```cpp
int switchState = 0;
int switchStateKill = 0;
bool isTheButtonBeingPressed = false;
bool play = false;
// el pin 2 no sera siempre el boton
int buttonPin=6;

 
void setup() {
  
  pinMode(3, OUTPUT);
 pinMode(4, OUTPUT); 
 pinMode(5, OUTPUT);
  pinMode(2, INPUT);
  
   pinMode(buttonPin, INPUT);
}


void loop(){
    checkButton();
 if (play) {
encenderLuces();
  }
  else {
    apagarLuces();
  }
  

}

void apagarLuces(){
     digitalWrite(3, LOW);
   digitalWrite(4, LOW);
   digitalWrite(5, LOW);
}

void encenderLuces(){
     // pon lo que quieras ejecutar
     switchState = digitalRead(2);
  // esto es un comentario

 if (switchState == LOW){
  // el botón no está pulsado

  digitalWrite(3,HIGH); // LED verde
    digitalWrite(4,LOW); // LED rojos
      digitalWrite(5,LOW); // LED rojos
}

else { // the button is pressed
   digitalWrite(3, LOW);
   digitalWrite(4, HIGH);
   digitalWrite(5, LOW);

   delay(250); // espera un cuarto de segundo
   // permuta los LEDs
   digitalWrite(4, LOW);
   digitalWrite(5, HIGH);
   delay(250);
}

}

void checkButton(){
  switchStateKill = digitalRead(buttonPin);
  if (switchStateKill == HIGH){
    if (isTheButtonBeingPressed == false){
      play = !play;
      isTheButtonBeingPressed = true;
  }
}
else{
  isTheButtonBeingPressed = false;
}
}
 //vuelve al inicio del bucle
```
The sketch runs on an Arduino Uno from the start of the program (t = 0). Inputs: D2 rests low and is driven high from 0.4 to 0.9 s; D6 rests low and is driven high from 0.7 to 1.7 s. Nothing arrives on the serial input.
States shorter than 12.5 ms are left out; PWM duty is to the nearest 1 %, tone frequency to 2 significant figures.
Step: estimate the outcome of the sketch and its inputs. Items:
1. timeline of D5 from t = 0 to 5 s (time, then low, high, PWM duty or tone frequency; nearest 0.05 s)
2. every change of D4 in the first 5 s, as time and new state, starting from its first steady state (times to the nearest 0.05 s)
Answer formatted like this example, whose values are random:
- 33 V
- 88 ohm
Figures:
- 0 s low; 0.95 s high; 1.2 s low
- 0 s low; 0.7 s high; 0.95 s low
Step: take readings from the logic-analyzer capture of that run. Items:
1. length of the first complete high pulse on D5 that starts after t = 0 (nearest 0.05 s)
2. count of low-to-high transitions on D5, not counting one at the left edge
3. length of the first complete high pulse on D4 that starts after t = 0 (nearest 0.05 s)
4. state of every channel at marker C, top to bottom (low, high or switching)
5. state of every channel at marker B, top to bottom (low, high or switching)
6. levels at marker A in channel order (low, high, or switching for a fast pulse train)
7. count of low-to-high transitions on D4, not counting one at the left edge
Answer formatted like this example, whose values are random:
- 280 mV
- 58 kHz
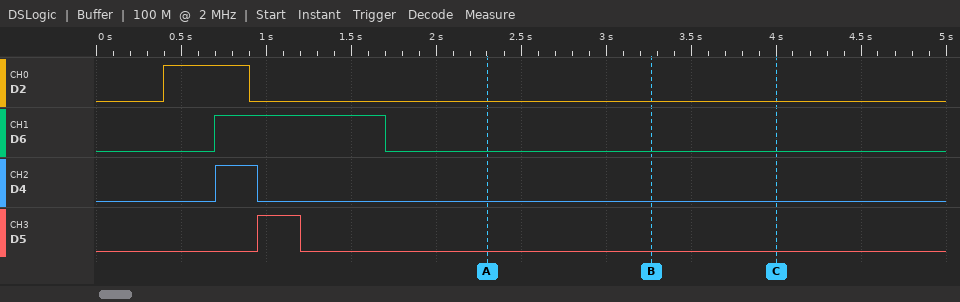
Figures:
- 0.25 s
- 1
- 0.25 s
- D2 low, D6 low, D4 low, D5 low
- D2 low, D6 low, D4 low, D5 low
- D2 low, D6 low, D4 low, D5 low
- 1
